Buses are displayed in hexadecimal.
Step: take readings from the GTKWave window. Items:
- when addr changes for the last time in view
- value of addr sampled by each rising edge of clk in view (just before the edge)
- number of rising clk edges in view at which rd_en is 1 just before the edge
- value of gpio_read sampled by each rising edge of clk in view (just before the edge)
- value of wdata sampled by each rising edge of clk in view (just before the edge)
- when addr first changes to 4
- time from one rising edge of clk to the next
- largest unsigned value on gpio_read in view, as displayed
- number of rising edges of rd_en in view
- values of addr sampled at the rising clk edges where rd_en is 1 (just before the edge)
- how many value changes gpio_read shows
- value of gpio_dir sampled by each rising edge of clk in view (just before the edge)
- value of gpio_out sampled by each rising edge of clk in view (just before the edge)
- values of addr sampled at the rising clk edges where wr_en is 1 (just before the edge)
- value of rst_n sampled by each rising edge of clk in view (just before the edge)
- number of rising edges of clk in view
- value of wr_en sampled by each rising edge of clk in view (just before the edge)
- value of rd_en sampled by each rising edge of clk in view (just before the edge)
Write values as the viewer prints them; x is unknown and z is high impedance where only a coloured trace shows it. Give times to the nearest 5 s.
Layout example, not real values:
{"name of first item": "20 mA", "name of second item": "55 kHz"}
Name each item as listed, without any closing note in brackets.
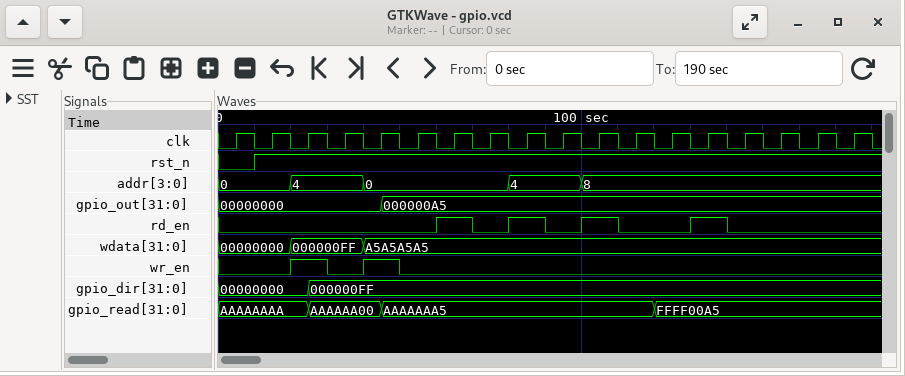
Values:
{"when addr changes for the last time in view": "100 s", "value of addr sampled by each rising edge of clk in view": "0, 0, 4, 4, 0, 0, 0, 0, 4, 4, 8, 8, 8, 8, 8, 8, 8, 8", "number of rising clk edges in view at which rd_en is 1 just before the edge": "4", "value of gpio_read sampled by each rising edge of clk in view": "AAAAAAAA, AAAAAAAA, AAAAAAAA, AAAAAA00, AAAAAA00, AAAAAAA5, AAAAAAA5, AAAAAAA5, AAAAAAA5, AAAAAAA5, AAAAAAA5, AAAAAAA5, FFFF00A5, FFFF00A5, FFFF00A5, FFFF00A5, FFFF00A5, FFFF00A5", "value of wdata sampled by each rising edge of clk in view": "00000000, 00000000, 000000FF, 000000FF, A5A5A5A5, A5A5A5A5, A5A5A5A5, A5A5A5A5, A5A5A5A5, A5A5A5A5, A5A5A5A5, A5A5A5A5, A5A5A5A5, A5A5A5A5, A5A5A5A5, A5A5A5A5, A5A5A5A5, A5A5A5A5", "when addr first changes to 4": "20 s", "time from one rising edge of clk to the next": "10 s", "largest unsigned value on gpio_read in view, as displayed": "FFFF00A5", "number of rising edges of rd_en in view": "4", "values of addr sampled at the rising clk edges where rd_en is 1": "0, 4, 8, 8", "how many value changes gpio_read shows": "3", "value of gpio_dir sampled by each rising edge of clk in view": "00000000, 00000000, 00000000, 000000FF, 000000FF, 000000FF, 000000FF, 000000FF, 000000FF, 000000FF, 000000FF, 000000FF, 000000FF, 000000FF, 000000FF, 000000FF, 000000FF, 000000FF", "value of gpio_out sampled by each rising edge of clk in view": "00000000, 00000000, 00000000, 00000000, 00000000, 000000A5, 000000A5, 000000A5, 000000A5, 000000A5, 000000A5, 000000A5, 000000A5, 000000A5, 000000A5, 000000A5, 000000A5, 000000A5", "values of addr sampled at the rising clk edges where wr_en is 1": "4, 0", "value of rst_n sampled by each rising edge of clk in view": "0 1 1 1 1 1 1 1 1 1 1 1 1 1 1 1 1 1", "number of rising edges of clk in view": "18", "value of wr_en sampled by each rising edge of clk in view": "0 0 1 0 1 0 0 0 0 0 0 0 0 0 0 0 0 0", "value of rd_en sampled by each rising edge of clk in view": "0 0 0 0 0 0 1 0 1 0 1 0 0 1 0 0 0 0"}
